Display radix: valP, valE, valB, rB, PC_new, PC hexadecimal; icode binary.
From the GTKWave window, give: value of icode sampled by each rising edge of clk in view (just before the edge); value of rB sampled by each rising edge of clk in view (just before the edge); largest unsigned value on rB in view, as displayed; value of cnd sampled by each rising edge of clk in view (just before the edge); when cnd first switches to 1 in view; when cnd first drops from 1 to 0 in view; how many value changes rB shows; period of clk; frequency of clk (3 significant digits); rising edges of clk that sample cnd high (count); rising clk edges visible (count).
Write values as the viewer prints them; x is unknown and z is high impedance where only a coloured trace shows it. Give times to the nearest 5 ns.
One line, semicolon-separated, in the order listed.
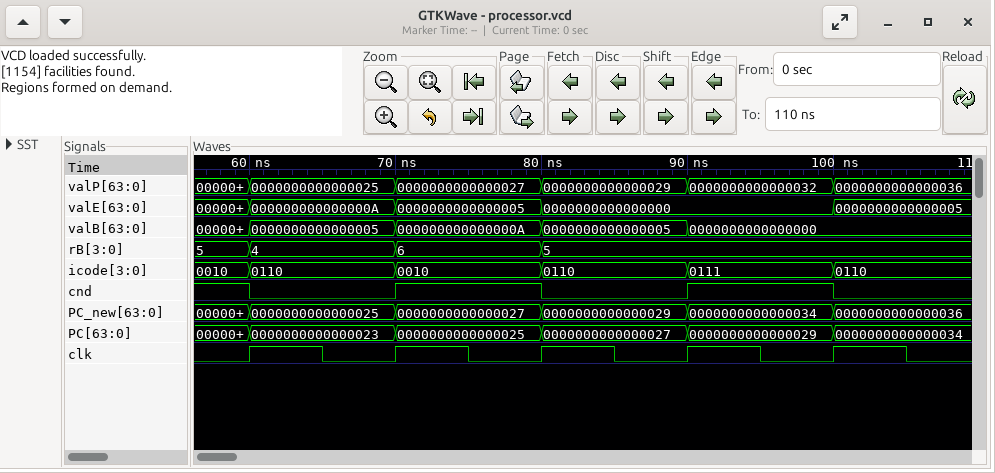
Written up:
0010, 0110, 0010, 0110, 0111; 5, 4, 6, 5, 5; 6; 1 0 1 0 1; 70 ns; 60 ns; 3; 10 ns; 100 MHz; 3; 5
